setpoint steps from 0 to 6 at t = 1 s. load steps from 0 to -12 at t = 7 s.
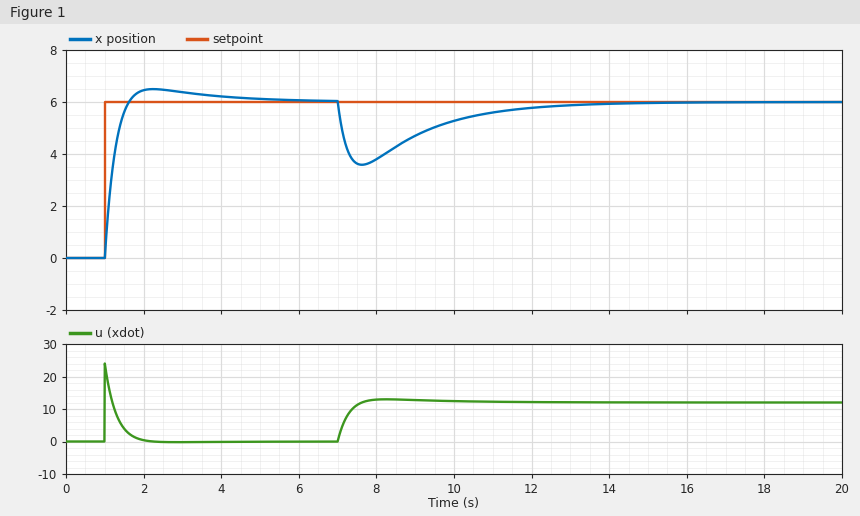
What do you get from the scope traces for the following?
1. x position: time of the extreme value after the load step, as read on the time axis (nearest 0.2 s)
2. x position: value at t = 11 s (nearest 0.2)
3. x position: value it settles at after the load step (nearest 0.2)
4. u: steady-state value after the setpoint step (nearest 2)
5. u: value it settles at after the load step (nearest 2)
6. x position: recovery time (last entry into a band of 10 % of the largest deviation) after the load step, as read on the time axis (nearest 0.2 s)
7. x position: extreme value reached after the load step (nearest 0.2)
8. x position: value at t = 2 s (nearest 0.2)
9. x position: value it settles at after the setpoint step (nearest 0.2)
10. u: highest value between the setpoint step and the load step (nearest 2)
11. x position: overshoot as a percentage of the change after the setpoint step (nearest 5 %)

7.6 s
5.6
6.0
0
12
11.8 s
3.6
6.4
6.0
24
10 %
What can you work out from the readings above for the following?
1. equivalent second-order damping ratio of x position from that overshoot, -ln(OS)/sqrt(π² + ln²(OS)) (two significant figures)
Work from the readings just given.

0.59
